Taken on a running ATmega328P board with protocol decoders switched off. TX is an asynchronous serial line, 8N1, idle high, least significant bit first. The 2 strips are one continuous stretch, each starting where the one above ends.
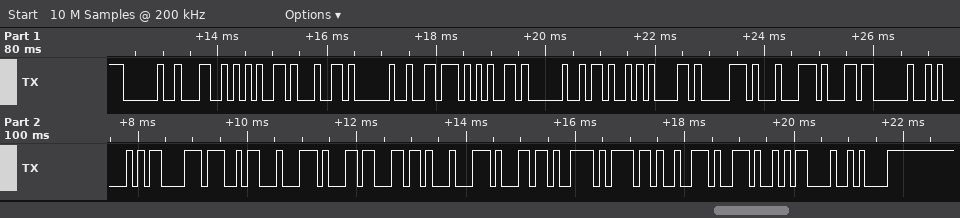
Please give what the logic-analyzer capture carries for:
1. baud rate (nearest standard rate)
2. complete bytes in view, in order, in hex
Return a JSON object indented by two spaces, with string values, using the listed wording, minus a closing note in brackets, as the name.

{
  "baud rate": "9600 baud",
  "complete bytes in view, in order, in hex": "20 4C 65 64 20 76 65 20 4B 61 70 C4 B1 20 41 C3 A7 C4 B1 6C C4 B1 79 6F 72 2E 0D 0A"
}
